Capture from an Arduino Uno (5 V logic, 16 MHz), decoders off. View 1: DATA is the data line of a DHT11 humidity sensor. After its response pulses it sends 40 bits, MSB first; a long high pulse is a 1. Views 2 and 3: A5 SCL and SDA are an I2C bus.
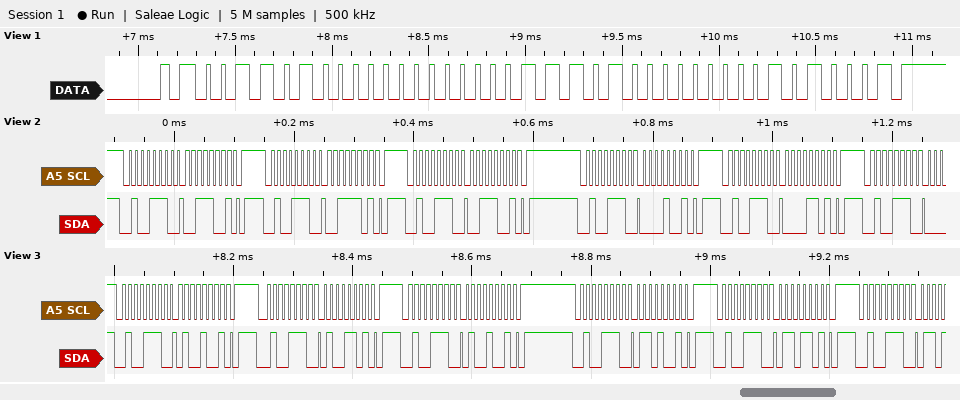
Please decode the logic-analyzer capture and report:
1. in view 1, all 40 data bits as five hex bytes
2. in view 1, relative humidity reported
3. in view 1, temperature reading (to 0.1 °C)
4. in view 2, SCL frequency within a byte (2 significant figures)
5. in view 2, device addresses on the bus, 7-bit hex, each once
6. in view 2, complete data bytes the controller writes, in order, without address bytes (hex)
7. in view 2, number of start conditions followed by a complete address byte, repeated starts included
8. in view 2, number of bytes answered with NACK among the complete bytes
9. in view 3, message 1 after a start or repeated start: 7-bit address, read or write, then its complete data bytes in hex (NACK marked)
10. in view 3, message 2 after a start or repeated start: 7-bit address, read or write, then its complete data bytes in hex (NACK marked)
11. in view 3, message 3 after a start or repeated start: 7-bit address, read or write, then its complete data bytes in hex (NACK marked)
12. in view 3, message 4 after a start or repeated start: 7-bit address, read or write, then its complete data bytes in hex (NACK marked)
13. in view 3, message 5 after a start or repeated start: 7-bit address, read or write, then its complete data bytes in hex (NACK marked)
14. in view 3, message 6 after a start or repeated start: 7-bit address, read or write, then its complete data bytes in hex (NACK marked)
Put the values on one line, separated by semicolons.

34 00 1D 00 51; 52 %; 29.0 °C; 100 kHz; 0x27; 39 3D 39 09 0D; 6; 0; 0x27 write: 49; 0x27 write: 4D; 0x27 write: 49; 0x27 write: 69; 0x27 write: 6D; 0x27 write
